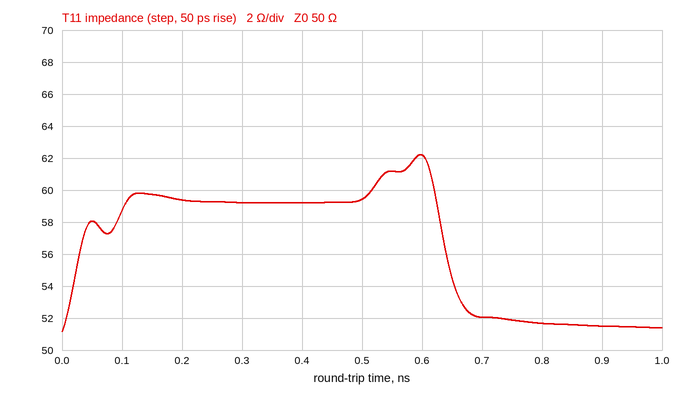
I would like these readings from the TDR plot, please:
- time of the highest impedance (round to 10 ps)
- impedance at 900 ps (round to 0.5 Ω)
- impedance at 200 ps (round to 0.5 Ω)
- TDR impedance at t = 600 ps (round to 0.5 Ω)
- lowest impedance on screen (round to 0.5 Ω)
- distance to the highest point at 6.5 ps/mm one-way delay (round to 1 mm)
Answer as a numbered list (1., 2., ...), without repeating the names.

1. 600 ps
2. 51.5 Ω
3. 59.5 Ω
4. 62.0 Ω
5. 51.0 Ω
6. 46 mm
